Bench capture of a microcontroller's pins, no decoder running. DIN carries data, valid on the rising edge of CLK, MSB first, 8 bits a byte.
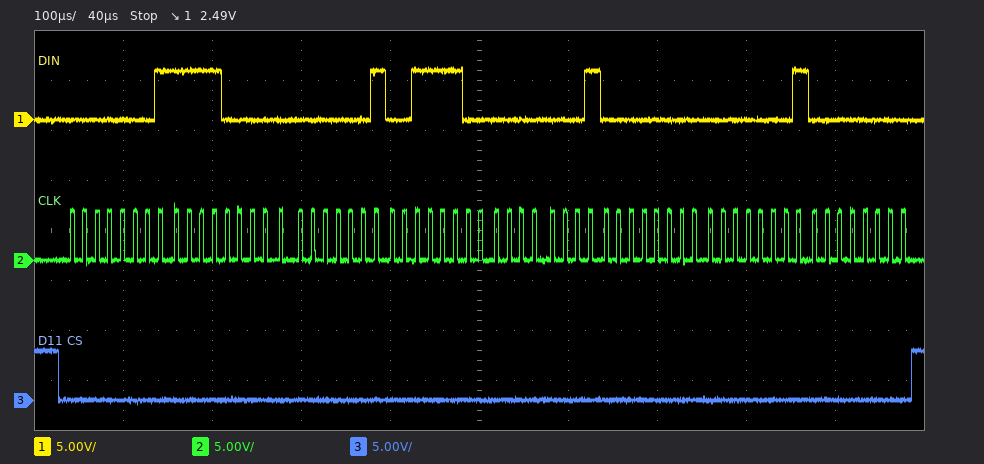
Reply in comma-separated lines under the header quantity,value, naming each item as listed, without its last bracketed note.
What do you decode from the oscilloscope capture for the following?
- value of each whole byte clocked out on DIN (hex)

quantity,value
value of each whole byte clocked out on DIN,0x01 0xF0 0x01 0x3C 0x01 0x00 0x01 0x00
